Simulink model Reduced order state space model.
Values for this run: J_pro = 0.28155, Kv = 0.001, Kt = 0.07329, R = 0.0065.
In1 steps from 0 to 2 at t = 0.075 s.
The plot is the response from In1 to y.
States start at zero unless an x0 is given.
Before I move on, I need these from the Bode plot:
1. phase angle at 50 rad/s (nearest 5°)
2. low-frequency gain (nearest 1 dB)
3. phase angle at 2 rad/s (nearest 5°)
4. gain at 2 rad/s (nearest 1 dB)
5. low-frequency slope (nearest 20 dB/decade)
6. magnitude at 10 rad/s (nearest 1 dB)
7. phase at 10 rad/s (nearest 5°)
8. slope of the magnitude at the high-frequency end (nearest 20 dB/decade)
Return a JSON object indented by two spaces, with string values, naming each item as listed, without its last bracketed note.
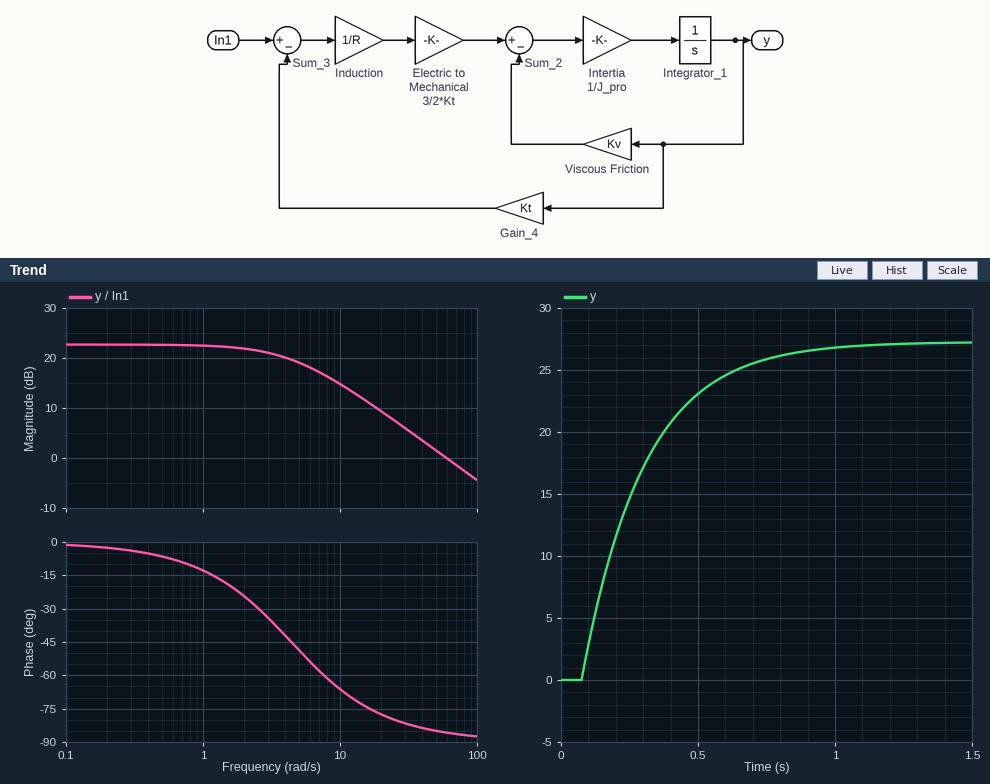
{
  "phase angle at 50 rad/s": "-85°",
  "low-frequency gain": "23 dB",
  "phase angle at 2 rad/s": "-25°",
  "gain at 2 rad/s": "22 dB",
  "low-frequency slope": "0 dB/decade",
  "magnitude at 10 rad/s": "15 dB",
  "phase at 10 rad/s": "-65°",
  "slope of the magnitude at the high-frequency end": "-20 dB/decade"
}
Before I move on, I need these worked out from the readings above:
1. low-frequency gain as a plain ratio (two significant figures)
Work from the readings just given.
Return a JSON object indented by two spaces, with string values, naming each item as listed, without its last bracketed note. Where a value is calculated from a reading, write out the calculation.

{
  "low-frequency gain as a plain ratio": "10^(23 / 20) = 14"
}
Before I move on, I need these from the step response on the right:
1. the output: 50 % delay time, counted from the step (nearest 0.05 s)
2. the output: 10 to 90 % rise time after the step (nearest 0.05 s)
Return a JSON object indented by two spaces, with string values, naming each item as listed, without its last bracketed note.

{
  "the output: 50 % delay time, counted from the step": "0.15 s",
  "the output: 10 to 90 % rise time after the step": "0.50 s"
}
